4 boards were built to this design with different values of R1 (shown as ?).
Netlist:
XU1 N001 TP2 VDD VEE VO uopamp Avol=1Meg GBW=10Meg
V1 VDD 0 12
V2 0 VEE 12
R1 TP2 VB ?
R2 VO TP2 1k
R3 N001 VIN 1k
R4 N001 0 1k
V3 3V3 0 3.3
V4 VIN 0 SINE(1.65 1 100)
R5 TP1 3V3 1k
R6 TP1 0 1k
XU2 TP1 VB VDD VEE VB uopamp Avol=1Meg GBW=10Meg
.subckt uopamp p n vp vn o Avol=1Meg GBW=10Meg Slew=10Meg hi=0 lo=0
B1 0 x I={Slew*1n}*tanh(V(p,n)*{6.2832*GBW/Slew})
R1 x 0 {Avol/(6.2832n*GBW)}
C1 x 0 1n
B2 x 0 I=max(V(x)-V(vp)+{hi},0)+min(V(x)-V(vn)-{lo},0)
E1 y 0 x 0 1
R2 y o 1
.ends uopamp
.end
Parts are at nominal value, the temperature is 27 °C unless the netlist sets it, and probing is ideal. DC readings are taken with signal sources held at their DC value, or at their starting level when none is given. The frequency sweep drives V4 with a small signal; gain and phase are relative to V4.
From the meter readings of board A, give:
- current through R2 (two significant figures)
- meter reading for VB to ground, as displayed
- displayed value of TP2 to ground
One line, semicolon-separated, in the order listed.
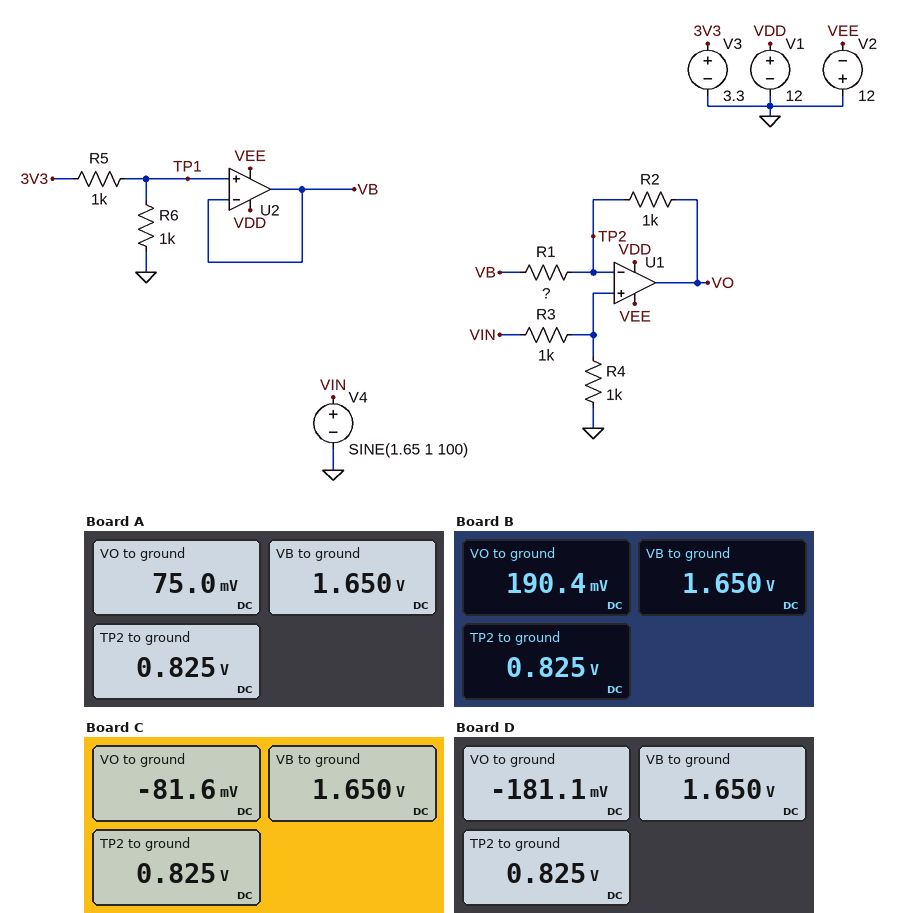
750 µA; 1.650 V; 0.825 V
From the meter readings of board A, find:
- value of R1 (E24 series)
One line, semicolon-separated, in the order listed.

1.1 kΩ
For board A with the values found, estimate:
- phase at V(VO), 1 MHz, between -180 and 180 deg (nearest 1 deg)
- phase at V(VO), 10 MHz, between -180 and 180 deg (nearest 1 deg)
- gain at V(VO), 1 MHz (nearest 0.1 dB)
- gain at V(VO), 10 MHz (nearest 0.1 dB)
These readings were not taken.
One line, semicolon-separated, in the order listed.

-11 deg; -62 deg; -0.6 dB; -7.1 dB
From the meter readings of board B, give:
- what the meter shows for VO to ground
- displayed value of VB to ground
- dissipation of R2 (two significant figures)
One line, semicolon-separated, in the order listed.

190.4 mV; 1.650 V; 400 µW
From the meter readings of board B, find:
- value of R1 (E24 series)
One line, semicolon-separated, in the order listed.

1.3 kΩ
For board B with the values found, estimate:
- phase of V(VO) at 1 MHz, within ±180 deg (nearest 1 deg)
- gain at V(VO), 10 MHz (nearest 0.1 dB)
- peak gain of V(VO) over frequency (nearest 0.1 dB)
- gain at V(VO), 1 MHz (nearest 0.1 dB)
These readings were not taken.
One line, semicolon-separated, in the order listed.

-10 deg; -7.2 dB; -1.1 dB; -1.2 dB
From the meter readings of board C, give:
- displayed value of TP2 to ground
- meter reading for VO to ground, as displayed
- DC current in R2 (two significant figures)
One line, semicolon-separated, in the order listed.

0.825 V; -81.6 mV; 910 µA
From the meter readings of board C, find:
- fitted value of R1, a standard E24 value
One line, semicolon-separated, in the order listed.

910 Ω
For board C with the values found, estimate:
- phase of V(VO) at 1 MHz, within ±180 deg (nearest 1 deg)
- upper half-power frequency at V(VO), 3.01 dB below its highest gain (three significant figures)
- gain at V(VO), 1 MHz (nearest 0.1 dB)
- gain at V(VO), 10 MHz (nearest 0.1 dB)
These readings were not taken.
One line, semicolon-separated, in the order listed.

-12 deg; 4.76 MHz; 0.2 dB; -6.9 dB
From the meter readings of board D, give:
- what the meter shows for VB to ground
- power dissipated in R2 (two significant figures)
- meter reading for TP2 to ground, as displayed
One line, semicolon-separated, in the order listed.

1.650 V; 1.0 mW; 0.825 V
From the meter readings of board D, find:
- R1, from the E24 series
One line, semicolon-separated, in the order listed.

820 Ω
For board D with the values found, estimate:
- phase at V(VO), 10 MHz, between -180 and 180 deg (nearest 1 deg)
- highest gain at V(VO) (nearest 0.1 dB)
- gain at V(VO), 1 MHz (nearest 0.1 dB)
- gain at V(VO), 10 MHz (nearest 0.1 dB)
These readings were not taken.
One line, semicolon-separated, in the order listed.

-66 deg; 0.9 dB; 0.7 dB; -6.8 dB
